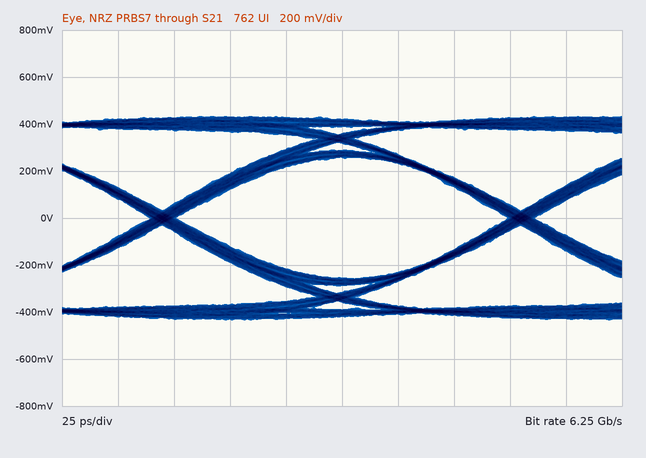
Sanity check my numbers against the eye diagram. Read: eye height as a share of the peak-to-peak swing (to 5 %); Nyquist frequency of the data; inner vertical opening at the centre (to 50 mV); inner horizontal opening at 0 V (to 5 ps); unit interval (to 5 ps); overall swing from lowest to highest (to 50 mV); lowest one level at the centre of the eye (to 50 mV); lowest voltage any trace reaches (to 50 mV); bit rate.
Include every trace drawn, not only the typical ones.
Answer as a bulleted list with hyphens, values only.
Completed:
- 60 %
- 3.125 GHz
- 500 mV
- 150 ps
- 160 ps
- 850 mV
- 250 mV
- -450 mV
- 6.25 Gb/s
